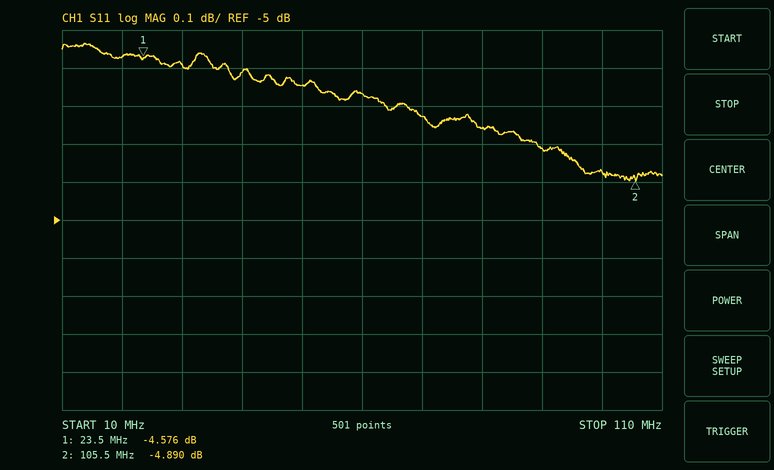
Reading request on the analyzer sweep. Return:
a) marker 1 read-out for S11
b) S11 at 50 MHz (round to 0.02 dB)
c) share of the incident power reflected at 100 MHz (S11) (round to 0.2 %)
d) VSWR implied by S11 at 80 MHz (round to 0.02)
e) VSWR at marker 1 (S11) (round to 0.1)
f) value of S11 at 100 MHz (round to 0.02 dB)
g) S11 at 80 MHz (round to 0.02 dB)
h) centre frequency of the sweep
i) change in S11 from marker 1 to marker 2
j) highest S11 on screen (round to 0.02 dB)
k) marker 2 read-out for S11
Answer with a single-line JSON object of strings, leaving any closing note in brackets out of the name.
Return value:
{"marker 1 read-out for S11": "-4.576 dB", "S11 at 50 MHz": "-4.64 dB", "share of the incident power reflected at 100 MHz (S11)": "32.6 %", "VSWR implied by S11 at 80 MHz": "3.74", "VSWR at marker 1 (S11)": "3.9", "value of S11 at 100 MHz": "-4.88 dB", "S11 at 80 MHz": "-4.76 dB", "centre frequency of the sweep": "60 MHz", "change in S11 from marker 1 to marker 2": "-0.314 dB", "highest S11 on screen": "-4.54 dB", "marker 2 read-out for S11": "-4.890 dB"}
